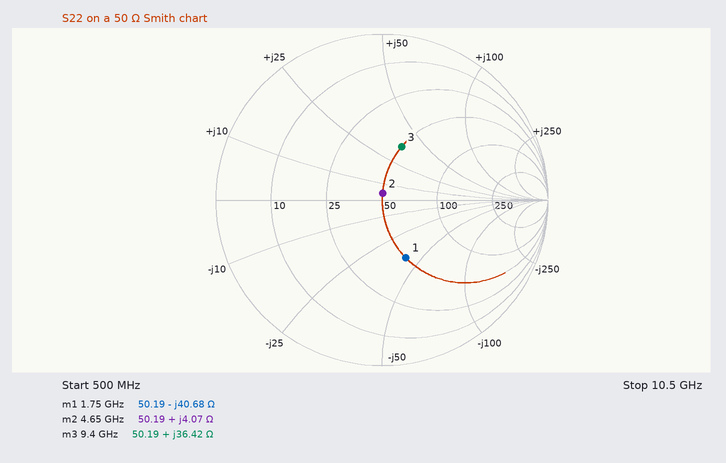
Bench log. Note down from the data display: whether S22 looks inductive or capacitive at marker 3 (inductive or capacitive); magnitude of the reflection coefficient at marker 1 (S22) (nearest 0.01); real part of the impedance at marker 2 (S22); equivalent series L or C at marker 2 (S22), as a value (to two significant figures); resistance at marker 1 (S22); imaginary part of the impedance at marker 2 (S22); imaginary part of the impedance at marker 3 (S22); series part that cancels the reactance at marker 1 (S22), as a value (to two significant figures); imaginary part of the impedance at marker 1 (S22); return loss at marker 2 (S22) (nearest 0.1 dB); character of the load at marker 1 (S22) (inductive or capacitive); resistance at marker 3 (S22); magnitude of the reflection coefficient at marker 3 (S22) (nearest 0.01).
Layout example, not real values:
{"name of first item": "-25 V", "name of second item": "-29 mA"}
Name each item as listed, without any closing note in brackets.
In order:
{"whether S22 looks inductive or capacitive at marker 3": "inductive", "magnitude of the reflection coefficient at marker 1 (S22)": "0.38", "real part of the impedance at marker 2": "50.19 Ω", "equivalent series L or C at marker 2 (S22), as a value": "140 pH", "resistance at marker 1": "50.19 Ω", "imaginary part of the impedance at marker 2": "+4.07 Ω", "imaginary part of the impedance at marker 3": "+36.42 Ω", "series part that cancels the reactance at marker 1 (S22), as a value": "3.7 nH", "imaginary part of the impedance at marker 1": "-40.68 Ω", "return loss at marker 2 (S22)": "27.8 dB", "character of the load at marker 1 (S22)": "capacitive", "resistance at marker 3": "50.19 Ω", "magnitude of the reflection coefficient at marker 3 (S22)": "0.34"}
